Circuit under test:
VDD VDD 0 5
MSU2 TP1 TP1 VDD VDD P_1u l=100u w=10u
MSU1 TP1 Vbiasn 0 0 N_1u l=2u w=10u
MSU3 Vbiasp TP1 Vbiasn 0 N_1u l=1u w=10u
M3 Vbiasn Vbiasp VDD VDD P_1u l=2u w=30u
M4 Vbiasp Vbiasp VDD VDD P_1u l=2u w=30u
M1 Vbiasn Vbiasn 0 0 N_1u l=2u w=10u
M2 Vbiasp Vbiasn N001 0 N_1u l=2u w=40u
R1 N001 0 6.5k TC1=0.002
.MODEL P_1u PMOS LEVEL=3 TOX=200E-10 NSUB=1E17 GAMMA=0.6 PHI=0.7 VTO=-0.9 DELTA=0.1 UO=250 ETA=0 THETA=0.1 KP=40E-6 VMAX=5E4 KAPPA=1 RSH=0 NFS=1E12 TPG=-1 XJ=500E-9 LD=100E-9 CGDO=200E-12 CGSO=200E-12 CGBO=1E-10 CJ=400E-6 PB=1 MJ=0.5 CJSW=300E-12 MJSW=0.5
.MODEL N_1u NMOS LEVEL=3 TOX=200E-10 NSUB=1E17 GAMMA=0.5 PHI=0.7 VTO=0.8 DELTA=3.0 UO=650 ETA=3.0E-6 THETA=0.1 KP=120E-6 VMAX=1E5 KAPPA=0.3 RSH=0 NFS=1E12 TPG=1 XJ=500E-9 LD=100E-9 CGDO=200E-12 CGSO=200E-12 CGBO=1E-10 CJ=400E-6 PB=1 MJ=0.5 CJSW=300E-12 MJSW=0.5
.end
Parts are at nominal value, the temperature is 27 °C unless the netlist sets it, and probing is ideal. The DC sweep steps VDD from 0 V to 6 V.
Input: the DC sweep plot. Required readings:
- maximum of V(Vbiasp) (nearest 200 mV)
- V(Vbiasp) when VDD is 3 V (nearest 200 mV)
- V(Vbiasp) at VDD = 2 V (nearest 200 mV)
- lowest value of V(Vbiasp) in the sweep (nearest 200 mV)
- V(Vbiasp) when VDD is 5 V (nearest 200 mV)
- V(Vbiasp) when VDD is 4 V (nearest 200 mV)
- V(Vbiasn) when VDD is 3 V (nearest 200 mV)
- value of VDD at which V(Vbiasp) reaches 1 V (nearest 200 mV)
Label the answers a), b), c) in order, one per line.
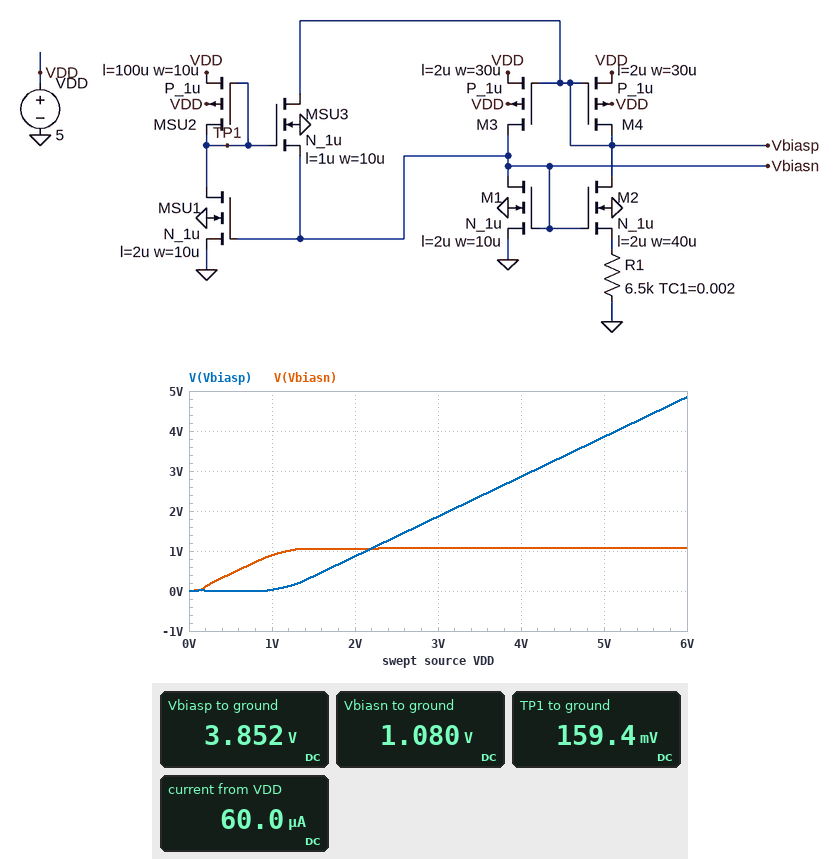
a) 4.8 V
b) 1.8 V
c) 800 mV
d) 0 V
e) 3.8 V
f) 2.8 V
g) 1.0 V
h) 2.2 V
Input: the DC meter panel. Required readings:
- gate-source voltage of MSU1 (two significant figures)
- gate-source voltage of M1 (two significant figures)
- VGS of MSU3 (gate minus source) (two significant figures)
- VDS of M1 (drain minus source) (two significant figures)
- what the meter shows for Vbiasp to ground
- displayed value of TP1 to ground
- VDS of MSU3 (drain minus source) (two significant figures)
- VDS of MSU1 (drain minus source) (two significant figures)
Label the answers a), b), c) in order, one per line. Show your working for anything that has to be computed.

a) 1.08 V = 1.1 V
b) 1.08 V = 1.1 V
c) 159.4 mV - 1.08 V = -920 mV
d) 1.08 V = 1.1 V
e) 3.852 V
f) 159.4 mV
g) 3.852 V - 1.08 V = 2.8 V
h) 159.4 mV = 160 mV
